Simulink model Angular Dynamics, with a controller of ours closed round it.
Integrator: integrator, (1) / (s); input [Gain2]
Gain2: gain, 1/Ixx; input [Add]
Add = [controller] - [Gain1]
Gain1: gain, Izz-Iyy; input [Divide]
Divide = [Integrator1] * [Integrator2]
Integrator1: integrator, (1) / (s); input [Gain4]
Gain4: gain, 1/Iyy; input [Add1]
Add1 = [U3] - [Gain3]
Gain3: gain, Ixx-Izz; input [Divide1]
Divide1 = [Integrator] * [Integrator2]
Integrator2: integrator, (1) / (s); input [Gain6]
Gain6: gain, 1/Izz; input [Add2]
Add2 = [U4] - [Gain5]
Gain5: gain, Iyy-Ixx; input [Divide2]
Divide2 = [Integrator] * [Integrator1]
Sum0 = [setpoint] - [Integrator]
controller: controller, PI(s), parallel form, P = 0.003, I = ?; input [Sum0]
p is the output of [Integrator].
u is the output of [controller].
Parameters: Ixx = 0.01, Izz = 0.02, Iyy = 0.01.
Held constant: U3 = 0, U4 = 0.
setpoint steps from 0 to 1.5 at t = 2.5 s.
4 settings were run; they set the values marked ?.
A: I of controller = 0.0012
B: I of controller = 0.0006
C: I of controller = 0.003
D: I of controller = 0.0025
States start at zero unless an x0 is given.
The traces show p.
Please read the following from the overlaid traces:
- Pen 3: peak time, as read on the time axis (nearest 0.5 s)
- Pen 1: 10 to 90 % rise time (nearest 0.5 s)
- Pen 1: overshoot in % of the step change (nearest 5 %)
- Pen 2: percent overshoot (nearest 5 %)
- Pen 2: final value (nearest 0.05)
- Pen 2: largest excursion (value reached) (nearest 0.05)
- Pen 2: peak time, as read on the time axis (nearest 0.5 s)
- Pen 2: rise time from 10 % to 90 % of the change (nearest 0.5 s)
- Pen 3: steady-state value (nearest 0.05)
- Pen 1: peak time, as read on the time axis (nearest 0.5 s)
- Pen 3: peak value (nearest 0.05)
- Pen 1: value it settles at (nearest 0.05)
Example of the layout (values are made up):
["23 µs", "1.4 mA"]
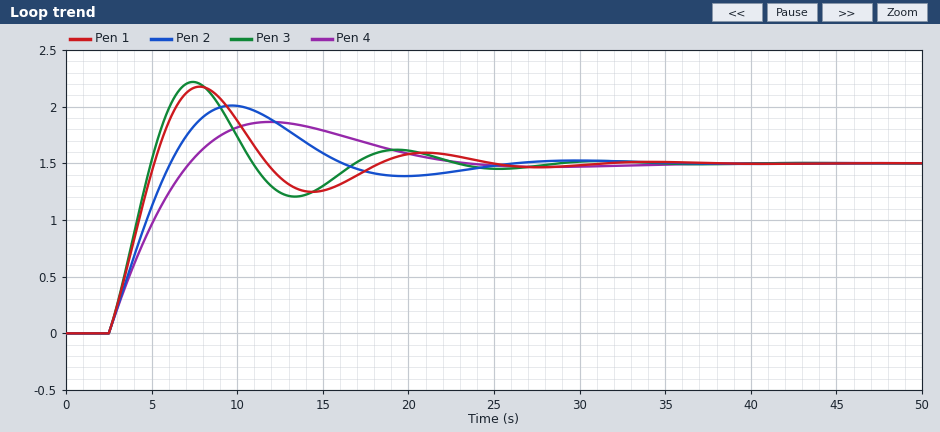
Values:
["7.5 s", "2.0 s", "45 %", "35 %", "1.50", "2.00", "9.5 s", "3.0 s", "1.50", "8.0 s", "2.20", "1.50"]
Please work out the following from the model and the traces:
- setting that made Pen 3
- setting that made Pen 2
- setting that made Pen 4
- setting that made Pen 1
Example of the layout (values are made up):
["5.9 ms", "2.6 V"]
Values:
["C", "A", "B", "D"]
